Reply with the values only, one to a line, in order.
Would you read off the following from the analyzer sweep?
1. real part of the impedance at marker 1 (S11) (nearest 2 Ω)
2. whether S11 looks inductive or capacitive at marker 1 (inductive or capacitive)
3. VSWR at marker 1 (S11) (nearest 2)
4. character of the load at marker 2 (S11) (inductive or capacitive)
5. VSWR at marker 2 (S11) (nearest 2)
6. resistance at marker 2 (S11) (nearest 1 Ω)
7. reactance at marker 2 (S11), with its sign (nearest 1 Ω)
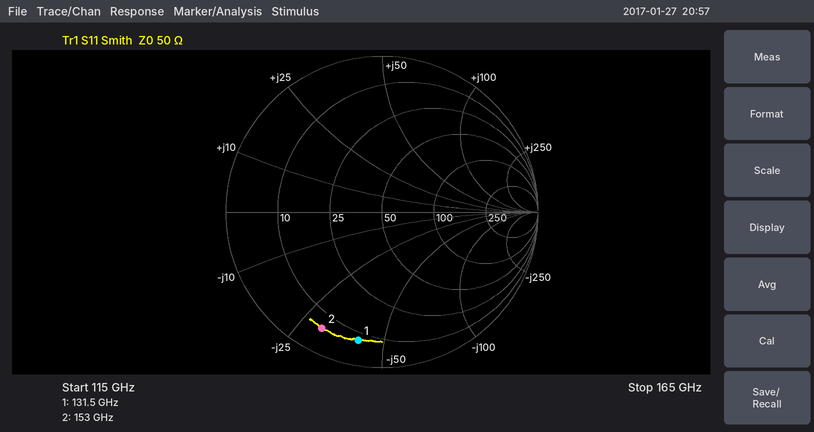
8 Ω
capacitive
12
capacitive
12
6 Ω
-30 Ω
